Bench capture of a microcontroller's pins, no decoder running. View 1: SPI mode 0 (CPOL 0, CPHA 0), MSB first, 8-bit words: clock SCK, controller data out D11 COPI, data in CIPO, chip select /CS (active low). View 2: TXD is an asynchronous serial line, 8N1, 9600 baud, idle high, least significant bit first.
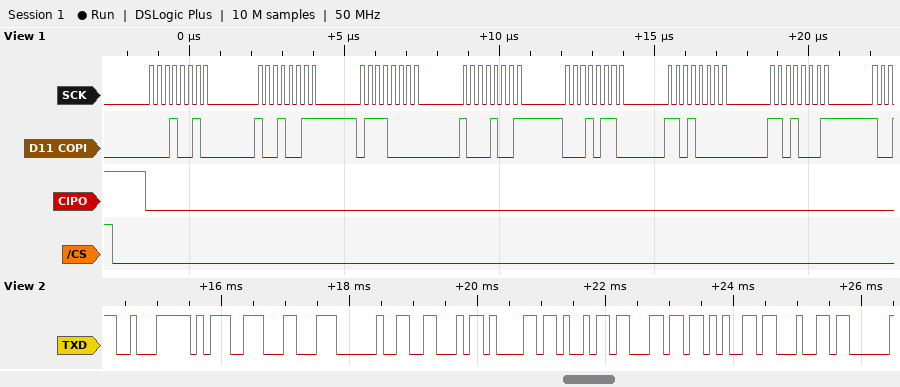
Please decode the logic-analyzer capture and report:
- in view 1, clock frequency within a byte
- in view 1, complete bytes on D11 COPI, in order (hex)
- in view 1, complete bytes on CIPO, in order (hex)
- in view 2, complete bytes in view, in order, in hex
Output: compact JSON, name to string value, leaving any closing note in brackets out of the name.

{"in view 1, clock frequency within a byte": "4 MHz", "in view 1, complete bytes on D11 COPI, in order": "12 93 70 89 16 D0 D1", "in view 1, complete bytes on CIPO, in order": "00 00 00 00 00 00 00", "in view 2, complete bytes in view, in order, in hex": "0xE2 0x9D 0x8C 0x20 0x46 0x61 0x69 0x6C 0x65 0x64"}
